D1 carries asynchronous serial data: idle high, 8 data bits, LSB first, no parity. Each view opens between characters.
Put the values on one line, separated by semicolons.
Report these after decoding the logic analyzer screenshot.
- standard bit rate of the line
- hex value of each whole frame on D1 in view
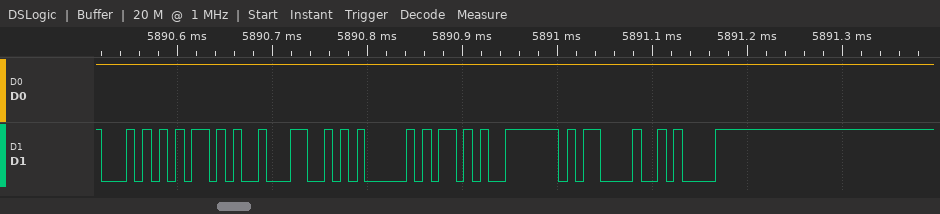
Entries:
115200 baud; 54, 2B, 4C, 41, 2B, 0D, 0A
